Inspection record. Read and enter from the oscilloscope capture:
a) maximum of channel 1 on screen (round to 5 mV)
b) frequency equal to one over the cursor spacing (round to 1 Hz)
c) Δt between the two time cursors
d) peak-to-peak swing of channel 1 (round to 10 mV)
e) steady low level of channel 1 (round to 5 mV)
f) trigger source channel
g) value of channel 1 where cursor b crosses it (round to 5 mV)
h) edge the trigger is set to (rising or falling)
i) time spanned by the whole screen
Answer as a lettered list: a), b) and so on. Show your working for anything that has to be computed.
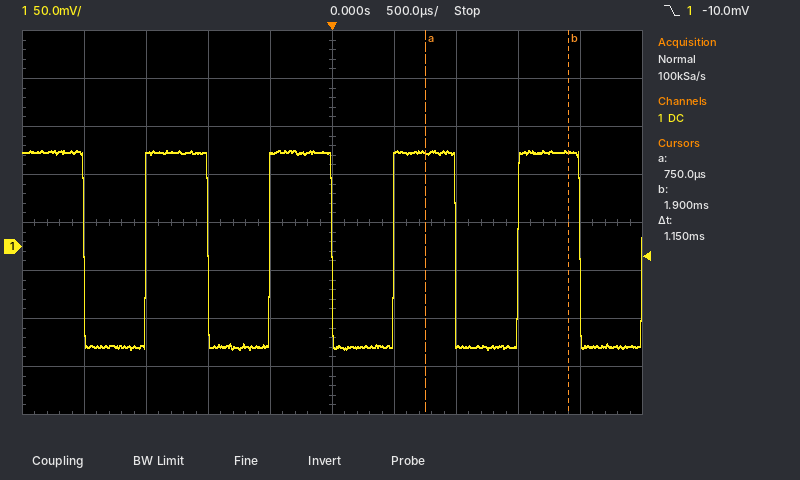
a) 100 mV
b) 1 / 1.15 ms ≈ 870 Hz
c) 1.15 ms
d) 210 mV
e) -105 mV
f) channel 1
g) 100 mV
h) falling
i) 5 ms
